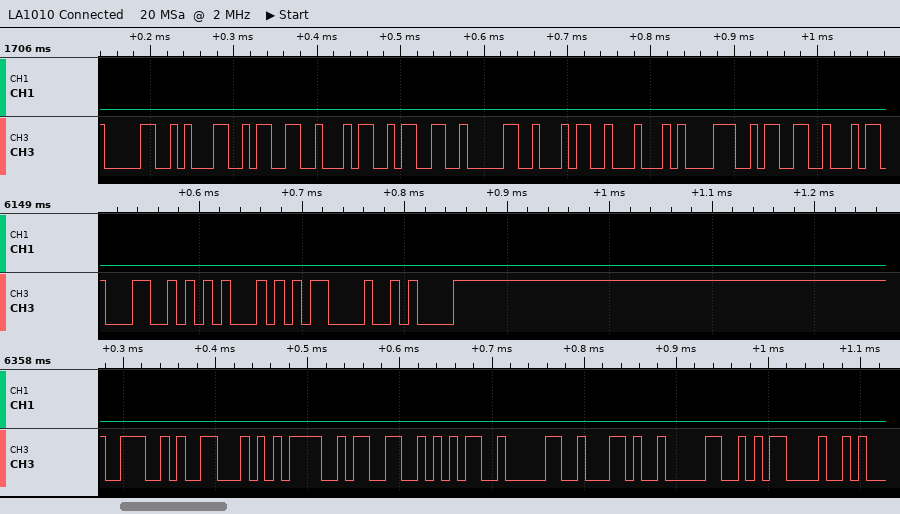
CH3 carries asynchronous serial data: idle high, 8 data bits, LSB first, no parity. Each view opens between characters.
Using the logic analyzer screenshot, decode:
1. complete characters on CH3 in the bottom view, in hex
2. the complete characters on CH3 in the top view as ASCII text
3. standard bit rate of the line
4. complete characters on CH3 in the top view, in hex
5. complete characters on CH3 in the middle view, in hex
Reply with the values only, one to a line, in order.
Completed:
4E, 46, 3D, 33, 35, 30, 2C, 30, 0D
"0134304D83"
115200 baud
30, 31, 33, 34, 33, 30, 34, 44, 38, 33
4C, 45, 0D, 0A
